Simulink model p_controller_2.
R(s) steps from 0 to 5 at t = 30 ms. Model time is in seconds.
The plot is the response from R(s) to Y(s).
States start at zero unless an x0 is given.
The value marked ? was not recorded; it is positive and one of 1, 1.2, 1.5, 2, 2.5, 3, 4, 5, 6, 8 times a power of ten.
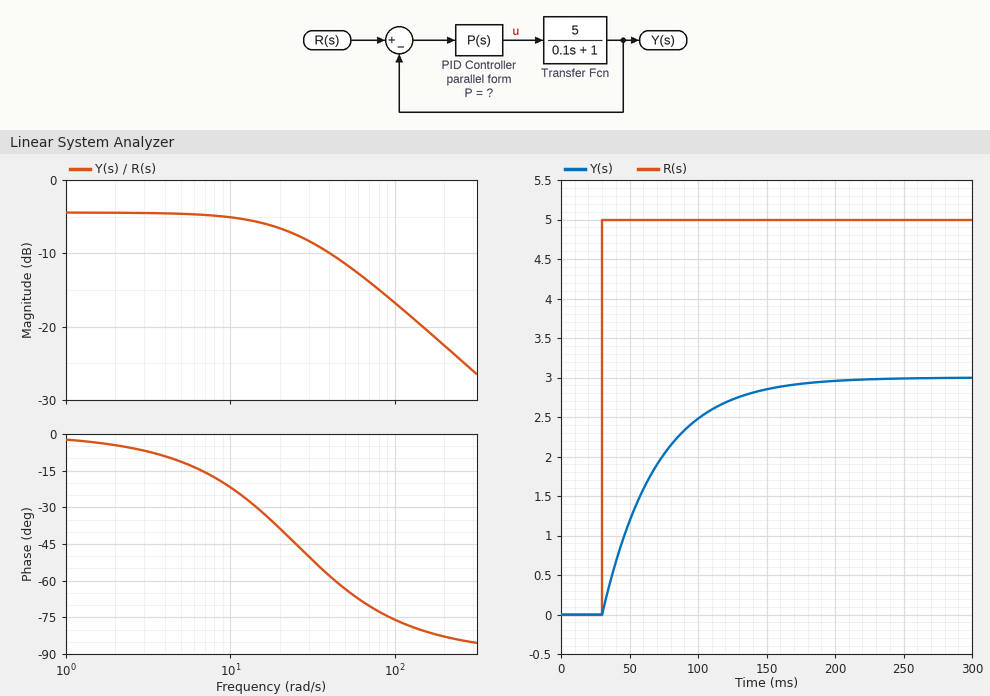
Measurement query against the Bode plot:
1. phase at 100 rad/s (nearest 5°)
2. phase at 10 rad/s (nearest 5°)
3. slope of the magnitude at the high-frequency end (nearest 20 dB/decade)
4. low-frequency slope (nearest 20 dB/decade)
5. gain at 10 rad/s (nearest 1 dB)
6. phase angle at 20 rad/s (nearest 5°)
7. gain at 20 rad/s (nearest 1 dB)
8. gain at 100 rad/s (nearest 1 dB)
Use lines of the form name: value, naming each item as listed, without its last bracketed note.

phase at 100 rad/s: -75°
phase at 10 rad/s: -20°
slope of the magnitude at the high-frequency end: -20 dB/decade
low-frequency slope: 0 dB/decade
gain at 10 rad/s: -5 dB
phase angle at 20 rad/s: -40°
gain at 20 rad/s: -7 dB
gain at 100 rad/s: -17 dB
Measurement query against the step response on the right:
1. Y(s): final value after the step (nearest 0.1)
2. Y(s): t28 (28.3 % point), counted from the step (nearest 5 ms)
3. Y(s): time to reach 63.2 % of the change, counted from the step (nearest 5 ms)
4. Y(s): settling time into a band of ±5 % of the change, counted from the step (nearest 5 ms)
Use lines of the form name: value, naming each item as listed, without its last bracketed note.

Y(s): final value after the step: 3.0
Y(s): t28 (28.3 % point), counted from the step: 15 ms
Y(s): time to reach 63.2 % of the change, counted from the step: 40 ms
Y(s): settling time into a band of ±5 % of the change, counted from the step: 120 ms
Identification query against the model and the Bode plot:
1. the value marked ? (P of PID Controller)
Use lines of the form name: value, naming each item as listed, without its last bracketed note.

the value marked ?: 0.3
